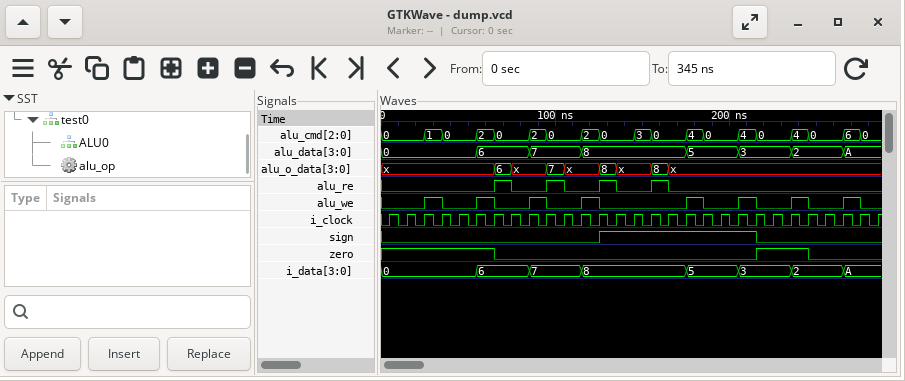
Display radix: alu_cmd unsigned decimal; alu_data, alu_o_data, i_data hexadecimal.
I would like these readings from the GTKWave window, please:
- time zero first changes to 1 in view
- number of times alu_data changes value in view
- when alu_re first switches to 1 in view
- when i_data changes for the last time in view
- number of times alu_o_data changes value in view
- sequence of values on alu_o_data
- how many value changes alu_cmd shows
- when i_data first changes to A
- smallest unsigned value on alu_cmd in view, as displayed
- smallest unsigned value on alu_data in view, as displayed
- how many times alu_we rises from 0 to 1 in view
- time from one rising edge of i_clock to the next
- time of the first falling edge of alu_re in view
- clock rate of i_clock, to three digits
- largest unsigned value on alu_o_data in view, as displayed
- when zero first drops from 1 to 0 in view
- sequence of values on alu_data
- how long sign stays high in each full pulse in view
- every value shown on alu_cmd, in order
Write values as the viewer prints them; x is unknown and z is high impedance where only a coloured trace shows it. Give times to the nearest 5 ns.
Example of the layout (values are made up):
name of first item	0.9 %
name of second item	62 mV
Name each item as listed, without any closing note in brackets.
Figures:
time zero first changes to 1 in view	215 ns
number of times alu_data changes value in view	7
when alu_re first switches to 1 in view	65 ns
when i_data changes for the last time in view	265 ns
number of times alu_o_data changes value in view	8
sequence of values on alu_o_data	x, 6, x, 7, x, 8, x, 8, x
how many value changes alu_cmd shows	18
when i_data first changes to A	265 ns
smallest unsigned value on alu_cmd in view, as displayed	0
smallest unsigned value on alu_data in view, as displayed	0
how many times alu_we rises from 0 to 1 in view	8
time from one rising edge of i_clock to the next	10 ns
time of the first falling edge of alu_re in view	75 ns
clock rate of i_clock, to three digits	100 MHz
largest unsigned value on alu_o_data in view, as displayed	8
when zero first drops from 1 to 0 in view	65 ns
sequence of values on alu_data	0, 6, 7, 8, 5, 3, 2, A
how long sign stays high in each full pulse in view	90 ns
every value shown on alu_cmd, in order	0, 1, 0, 2, 0, 2, 0, 2, 0, 3, 0, 4, 0, 4, 0, 4, 0, 6, 0
